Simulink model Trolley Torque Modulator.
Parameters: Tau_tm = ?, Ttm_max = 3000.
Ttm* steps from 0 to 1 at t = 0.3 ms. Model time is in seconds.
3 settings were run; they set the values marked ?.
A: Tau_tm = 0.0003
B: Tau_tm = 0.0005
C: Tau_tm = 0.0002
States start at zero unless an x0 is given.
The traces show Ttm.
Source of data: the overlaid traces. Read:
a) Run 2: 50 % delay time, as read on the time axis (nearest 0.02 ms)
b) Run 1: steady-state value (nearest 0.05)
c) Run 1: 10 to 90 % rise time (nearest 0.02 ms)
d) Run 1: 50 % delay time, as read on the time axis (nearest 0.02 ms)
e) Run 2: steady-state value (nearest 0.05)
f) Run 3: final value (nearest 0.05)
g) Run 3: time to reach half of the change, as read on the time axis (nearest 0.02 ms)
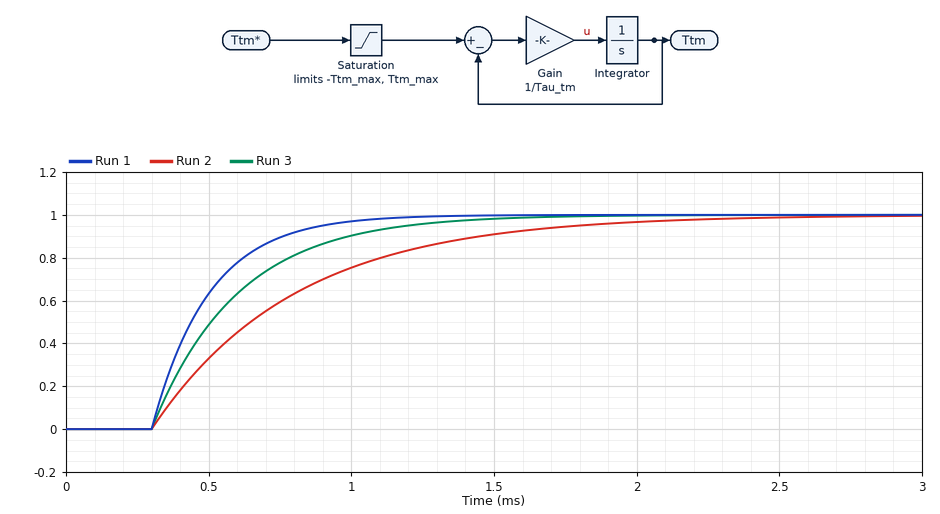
0.64 ms
1.00
0.44 ms
0.44 ms
1.00
1.00
0.50 ms
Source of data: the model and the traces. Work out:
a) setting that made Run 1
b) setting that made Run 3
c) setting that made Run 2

C
A
B
